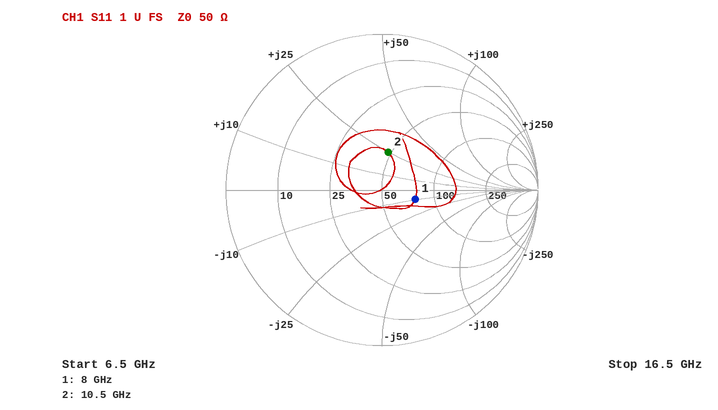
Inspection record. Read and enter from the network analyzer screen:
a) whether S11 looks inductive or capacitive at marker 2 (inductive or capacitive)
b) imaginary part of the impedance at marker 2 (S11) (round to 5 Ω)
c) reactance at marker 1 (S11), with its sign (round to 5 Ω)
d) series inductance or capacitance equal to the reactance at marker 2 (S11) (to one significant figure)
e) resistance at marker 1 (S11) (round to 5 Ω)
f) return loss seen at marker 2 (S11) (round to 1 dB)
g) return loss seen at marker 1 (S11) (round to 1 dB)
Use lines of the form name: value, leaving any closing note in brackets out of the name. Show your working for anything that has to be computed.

whether S11 looks inductive or capacitive at marker 2: inductive
imaginary part of the impedance at marker 2 (S11): +25 Ω
reactance at marker 1 (S11), with its sign: -10 Ω
series inductance or capacitance equal to the reactance at marker 2 (S11): L = 25 Ω/(2π × 10.5 GHz) ≈ 379 pH, so 400 pH to one significant figure
resistance at marker 1 (S11): 75 Ω
return loss seen at marker 2 (S11): 12 dB
return loss seen at marker 1 (S11): 13 dB
